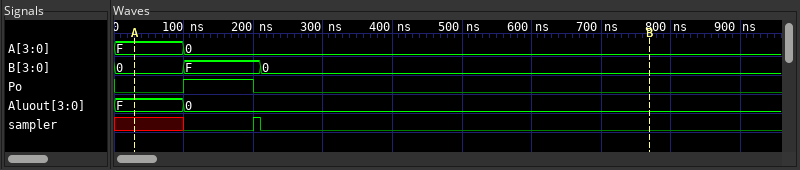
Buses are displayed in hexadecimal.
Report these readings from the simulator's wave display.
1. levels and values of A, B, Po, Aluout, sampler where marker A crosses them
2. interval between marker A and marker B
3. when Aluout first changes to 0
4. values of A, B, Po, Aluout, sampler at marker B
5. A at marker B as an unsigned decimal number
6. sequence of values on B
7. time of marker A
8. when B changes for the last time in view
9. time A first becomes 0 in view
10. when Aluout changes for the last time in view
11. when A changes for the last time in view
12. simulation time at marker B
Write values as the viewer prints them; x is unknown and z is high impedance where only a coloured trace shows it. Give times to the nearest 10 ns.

A=F, B=0, Po=0, Aluout=F, sampler=x
740 ns
100 ns
A=0, B=0, Po=0, Aluout=0, sampler=0
0
0, F, 0
30 ns
210 ns
100 ns
100 ns
100 ns
770 ns
